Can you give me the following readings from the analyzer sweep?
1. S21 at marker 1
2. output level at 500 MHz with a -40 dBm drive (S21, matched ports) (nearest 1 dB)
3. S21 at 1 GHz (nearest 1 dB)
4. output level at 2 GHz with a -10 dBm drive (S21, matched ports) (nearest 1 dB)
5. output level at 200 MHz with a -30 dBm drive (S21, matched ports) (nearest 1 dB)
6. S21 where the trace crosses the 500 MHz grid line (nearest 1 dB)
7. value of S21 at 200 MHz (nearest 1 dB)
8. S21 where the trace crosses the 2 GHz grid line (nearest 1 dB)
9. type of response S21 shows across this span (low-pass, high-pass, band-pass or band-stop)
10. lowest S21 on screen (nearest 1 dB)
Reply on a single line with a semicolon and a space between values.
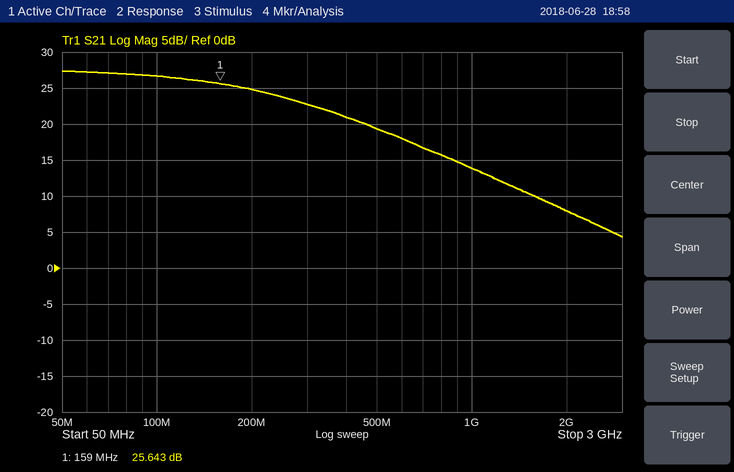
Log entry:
25.643 dB; -21 dBm; 14 dB; -2 dBm; -5 dBm; 19 dB; 25 dB; 8 dB; low-pass; 4 dB
